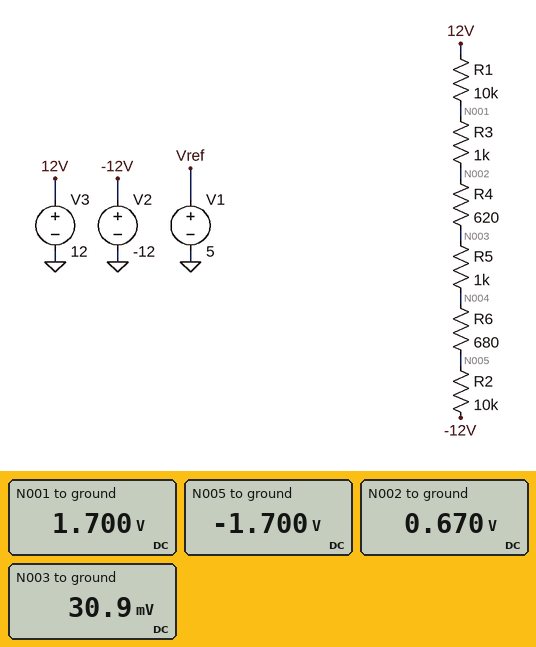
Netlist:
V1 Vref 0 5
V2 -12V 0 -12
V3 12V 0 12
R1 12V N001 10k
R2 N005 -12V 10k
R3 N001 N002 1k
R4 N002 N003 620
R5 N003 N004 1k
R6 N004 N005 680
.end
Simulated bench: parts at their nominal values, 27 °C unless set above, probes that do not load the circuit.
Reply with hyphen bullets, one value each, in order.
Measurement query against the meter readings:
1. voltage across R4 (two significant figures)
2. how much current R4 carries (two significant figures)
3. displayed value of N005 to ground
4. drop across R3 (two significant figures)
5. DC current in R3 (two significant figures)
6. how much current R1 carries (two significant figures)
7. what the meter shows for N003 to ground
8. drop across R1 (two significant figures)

- 640 mV
- 1.0 mA
- -1.700 V
- 1.0 V
- 1.0 mA
- 1.0 mA
- 30.9 mV
- 10 V
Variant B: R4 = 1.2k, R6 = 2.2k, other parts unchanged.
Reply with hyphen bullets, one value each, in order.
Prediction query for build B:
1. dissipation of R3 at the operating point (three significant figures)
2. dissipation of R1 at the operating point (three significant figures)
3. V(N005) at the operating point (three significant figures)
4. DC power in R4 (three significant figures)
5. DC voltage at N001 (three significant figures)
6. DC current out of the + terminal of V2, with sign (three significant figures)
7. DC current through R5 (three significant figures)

- 893 µW
- 8.93 mW
- -2.55 V
- 1.07 mW
- 2.55 V
- -945 µA
- 945 µA
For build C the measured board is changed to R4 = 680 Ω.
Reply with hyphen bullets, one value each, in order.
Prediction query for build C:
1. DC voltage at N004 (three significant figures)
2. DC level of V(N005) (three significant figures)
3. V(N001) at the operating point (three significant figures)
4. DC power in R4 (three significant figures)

- -1.03 V
- -1.73 V
- 1.73 V
- 718 µW
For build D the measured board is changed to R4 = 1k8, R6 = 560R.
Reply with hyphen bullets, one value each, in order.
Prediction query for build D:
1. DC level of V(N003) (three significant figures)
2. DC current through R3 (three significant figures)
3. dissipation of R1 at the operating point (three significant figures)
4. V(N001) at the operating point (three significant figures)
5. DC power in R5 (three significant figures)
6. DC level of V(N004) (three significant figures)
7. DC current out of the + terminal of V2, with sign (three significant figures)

- -611 mV
- 985 µA
- 9.71 mW
- 2.15 V
- 971 µW
- -1.60 V
- -985 µA
